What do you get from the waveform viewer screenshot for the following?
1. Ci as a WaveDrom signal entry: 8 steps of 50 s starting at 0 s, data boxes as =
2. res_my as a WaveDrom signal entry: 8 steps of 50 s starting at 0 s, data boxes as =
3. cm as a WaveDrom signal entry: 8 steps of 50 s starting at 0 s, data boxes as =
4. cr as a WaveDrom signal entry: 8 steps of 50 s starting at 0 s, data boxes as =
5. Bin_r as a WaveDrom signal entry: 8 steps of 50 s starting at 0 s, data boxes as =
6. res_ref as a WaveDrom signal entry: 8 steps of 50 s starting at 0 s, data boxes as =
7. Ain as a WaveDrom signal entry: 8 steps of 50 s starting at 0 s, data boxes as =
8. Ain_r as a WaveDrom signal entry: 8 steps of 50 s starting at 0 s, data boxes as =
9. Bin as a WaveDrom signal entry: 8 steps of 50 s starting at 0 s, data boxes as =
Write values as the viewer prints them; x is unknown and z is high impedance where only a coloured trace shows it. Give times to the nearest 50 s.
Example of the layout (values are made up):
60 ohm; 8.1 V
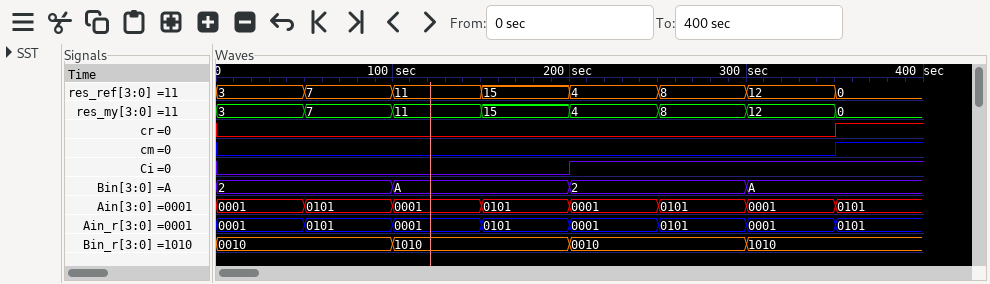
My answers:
{name: 'Ci', wave: '0...1...'}; {name: 'res_my', wave: '========', data: '3 7 11 15 4 8 12 0'}; {name: 'cm', wave: '0......1'}; {name: 'cr', wave: '0......1'}; {name: 'Bin_r', wave: '=.=.=.=.', data: '0010 1010 0010 1010'}; {name: 'res_ref', wave: '========', data: '3 7 11 15 4 8 12 0'}; {name: 'Ain', wave: '========', data: '0001 0101 0001 0101 0001 0101 0001 0101'}; {name: 'Ain_r', wave: '========', data: '0001 0101 0001 0101 0001 0101 0001 0101'}; {name: 'Bin', wave: '=.=.=.=.', data: '2 A 2 A'}
